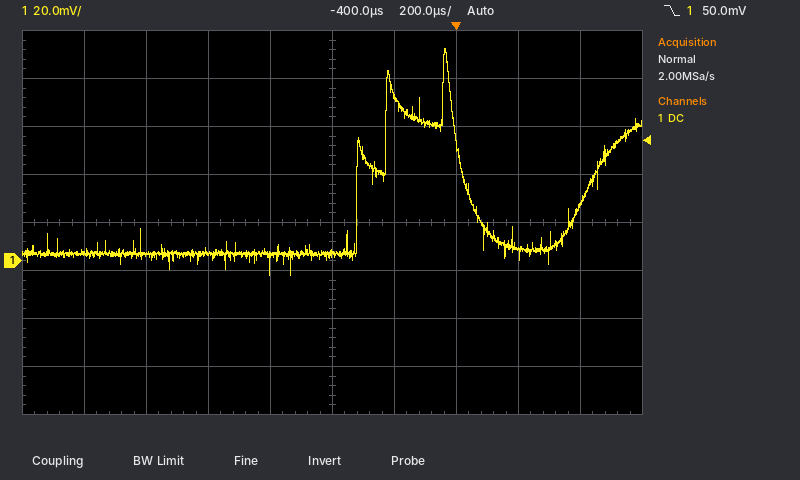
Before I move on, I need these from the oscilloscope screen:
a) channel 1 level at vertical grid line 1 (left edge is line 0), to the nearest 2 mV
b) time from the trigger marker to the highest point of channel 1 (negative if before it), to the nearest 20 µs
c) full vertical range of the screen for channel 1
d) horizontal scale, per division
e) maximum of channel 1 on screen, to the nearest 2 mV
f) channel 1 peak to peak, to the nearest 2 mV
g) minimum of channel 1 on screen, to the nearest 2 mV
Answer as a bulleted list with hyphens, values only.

- 4 mV
- -40 µs
- 160 mV
- 200 µs
- 88 mV
- 94 mV
- -6 mV
